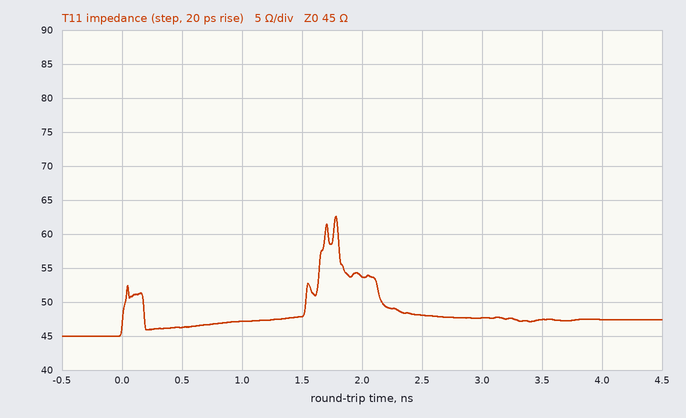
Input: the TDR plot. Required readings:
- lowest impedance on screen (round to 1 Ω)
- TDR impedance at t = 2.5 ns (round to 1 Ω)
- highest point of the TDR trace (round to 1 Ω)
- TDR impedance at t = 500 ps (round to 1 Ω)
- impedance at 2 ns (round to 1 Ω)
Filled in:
45 Ω
48 Ω
63 Ω
46 Ω
54 Ω
